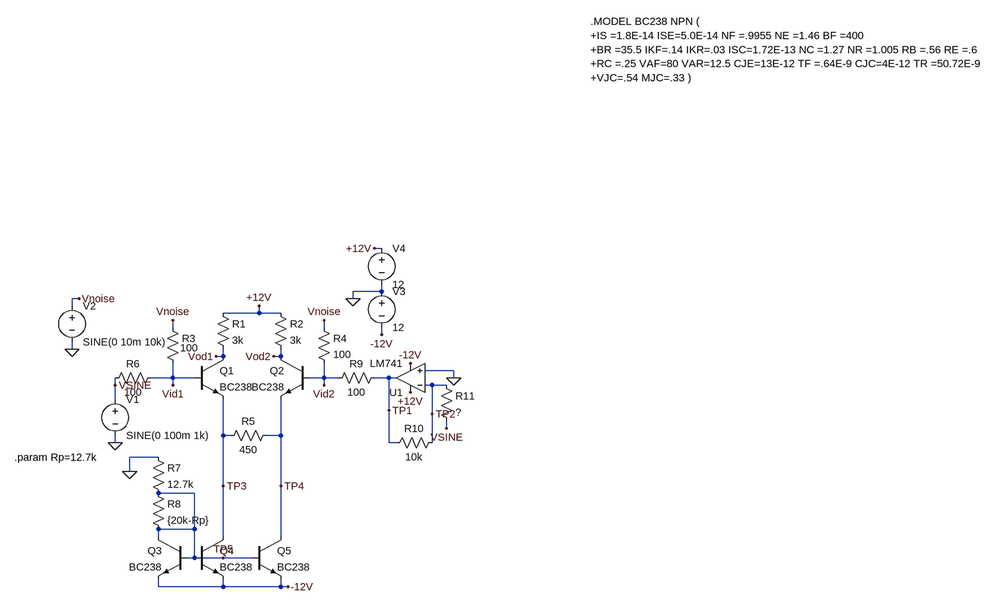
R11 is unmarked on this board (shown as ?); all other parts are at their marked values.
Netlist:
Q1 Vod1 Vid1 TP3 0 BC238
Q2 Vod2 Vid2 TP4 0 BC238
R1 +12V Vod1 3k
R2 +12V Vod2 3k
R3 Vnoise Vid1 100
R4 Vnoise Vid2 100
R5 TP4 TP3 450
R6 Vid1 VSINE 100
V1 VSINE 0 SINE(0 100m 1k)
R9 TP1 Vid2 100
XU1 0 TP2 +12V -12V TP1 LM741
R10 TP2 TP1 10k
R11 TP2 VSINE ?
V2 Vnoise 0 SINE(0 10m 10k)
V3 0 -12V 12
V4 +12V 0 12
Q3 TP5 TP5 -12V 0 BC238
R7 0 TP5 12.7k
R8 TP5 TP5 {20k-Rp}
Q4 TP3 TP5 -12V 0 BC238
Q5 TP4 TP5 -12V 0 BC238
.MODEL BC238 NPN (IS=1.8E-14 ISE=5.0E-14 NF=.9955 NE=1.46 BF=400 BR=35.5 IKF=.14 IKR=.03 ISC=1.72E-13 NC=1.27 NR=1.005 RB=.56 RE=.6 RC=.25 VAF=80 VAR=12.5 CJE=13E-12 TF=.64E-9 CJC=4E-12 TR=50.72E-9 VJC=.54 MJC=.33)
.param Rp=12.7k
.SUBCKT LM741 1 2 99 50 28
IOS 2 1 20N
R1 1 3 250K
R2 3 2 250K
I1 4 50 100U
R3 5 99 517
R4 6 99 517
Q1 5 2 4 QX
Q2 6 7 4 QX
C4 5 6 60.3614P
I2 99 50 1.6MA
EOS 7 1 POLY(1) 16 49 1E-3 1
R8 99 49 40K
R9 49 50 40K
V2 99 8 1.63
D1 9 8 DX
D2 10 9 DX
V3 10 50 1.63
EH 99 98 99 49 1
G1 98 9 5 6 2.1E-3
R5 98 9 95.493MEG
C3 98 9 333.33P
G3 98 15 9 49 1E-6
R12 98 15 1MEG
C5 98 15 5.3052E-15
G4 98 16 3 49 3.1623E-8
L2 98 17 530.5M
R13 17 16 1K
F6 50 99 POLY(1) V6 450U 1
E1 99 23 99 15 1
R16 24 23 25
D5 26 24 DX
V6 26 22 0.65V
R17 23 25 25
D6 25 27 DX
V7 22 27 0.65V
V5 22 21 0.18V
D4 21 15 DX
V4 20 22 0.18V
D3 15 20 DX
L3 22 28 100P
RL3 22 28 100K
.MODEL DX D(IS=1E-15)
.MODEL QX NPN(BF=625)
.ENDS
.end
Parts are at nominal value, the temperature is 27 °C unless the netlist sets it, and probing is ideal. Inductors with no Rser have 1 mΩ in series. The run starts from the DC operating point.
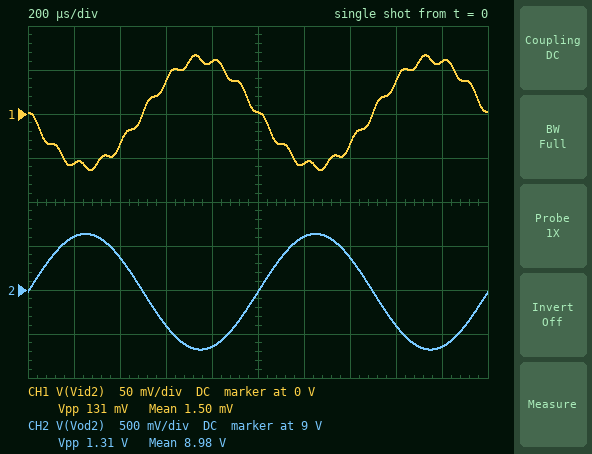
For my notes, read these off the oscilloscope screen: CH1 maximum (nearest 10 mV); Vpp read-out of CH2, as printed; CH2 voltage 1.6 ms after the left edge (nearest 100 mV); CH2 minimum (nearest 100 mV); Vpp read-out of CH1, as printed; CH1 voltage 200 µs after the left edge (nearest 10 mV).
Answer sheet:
70 mV
1.31 V
8.6 V
8.3 V
131 mV
-60 mV
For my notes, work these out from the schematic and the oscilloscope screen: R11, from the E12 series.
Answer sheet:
8.2 kΩ
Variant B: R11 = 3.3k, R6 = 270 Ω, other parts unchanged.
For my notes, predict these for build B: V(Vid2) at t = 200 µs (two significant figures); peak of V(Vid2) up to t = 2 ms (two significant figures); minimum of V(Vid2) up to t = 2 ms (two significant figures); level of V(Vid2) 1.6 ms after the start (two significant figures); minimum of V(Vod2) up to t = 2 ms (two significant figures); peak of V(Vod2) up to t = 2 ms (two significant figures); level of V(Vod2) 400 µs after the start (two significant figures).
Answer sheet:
-140 mV
160 mV
-150 mV
91 mV
7.9 V
10 V
9.6 V
